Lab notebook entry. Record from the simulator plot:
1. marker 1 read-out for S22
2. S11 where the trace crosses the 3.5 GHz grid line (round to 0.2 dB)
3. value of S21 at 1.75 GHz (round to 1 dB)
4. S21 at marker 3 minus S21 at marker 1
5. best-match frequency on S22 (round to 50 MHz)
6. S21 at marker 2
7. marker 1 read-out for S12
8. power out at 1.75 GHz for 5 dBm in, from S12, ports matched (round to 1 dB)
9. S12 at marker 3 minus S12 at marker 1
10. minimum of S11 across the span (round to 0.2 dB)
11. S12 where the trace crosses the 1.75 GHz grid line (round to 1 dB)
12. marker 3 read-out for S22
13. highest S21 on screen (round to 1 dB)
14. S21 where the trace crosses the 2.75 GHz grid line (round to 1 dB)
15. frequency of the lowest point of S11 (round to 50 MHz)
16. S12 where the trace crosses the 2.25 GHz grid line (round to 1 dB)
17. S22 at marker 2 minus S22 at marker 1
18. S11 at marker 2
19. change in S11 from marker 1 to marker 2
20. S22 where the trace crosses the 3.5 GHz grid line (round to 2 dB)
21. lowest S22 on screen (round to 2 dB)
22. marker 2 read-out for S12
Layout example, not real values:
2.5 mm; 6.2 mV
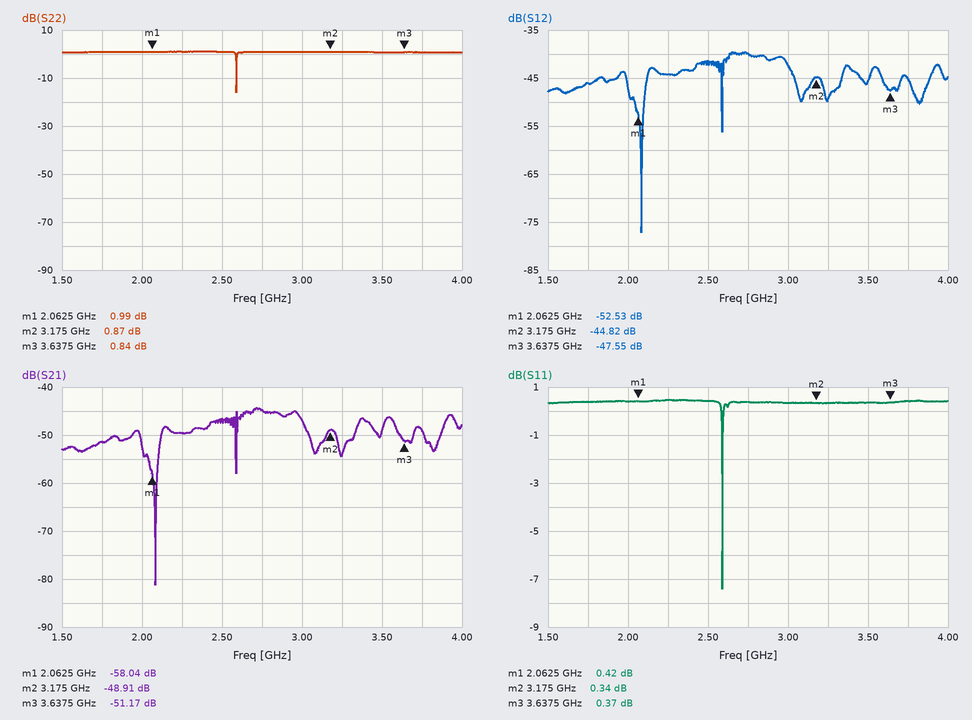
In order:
0.99 dB; 0.4 dB; -51 dB; 6.87 dB; 2.60 GHz; -48.91 dB; -52.53 dB; -41 dBm; 4.98 dB; -7.4 dB; -46 dB; 0.84 dB; -44 dB; -45 dB; 2.60 GHz; -44 dB; -0.12 dB; 0.34 dB; -0.08 dB; 0 dB; -16 dB; -44.82 dB
